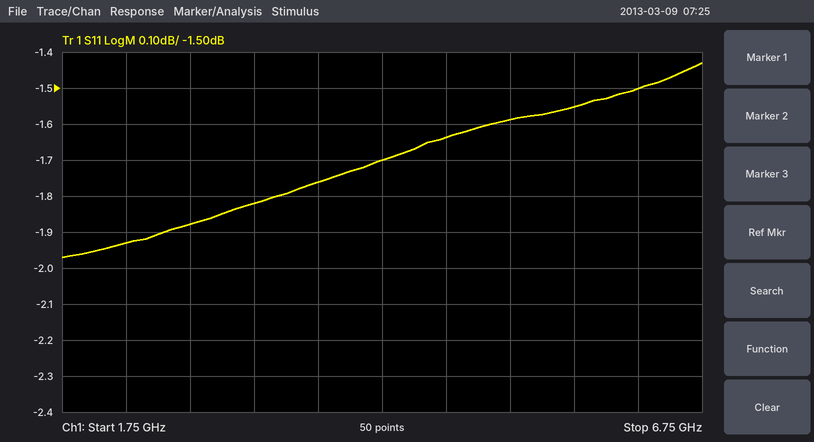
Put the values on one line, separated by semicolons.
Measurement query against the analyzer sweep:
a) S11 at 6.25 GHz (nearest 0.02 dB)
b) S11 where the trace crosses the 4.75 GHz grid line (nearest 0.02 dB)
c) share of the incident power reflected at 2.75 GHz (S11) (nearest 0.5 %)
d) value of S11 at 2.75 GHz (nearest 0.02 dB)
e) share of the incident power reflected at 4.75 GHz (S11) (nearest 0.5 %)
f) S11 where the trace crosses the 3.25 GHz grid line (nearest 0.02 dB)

-1.50 dB; -1.64 dB; 65.0 %; -1.88 dB; 68.5 %; -1.82 dB
